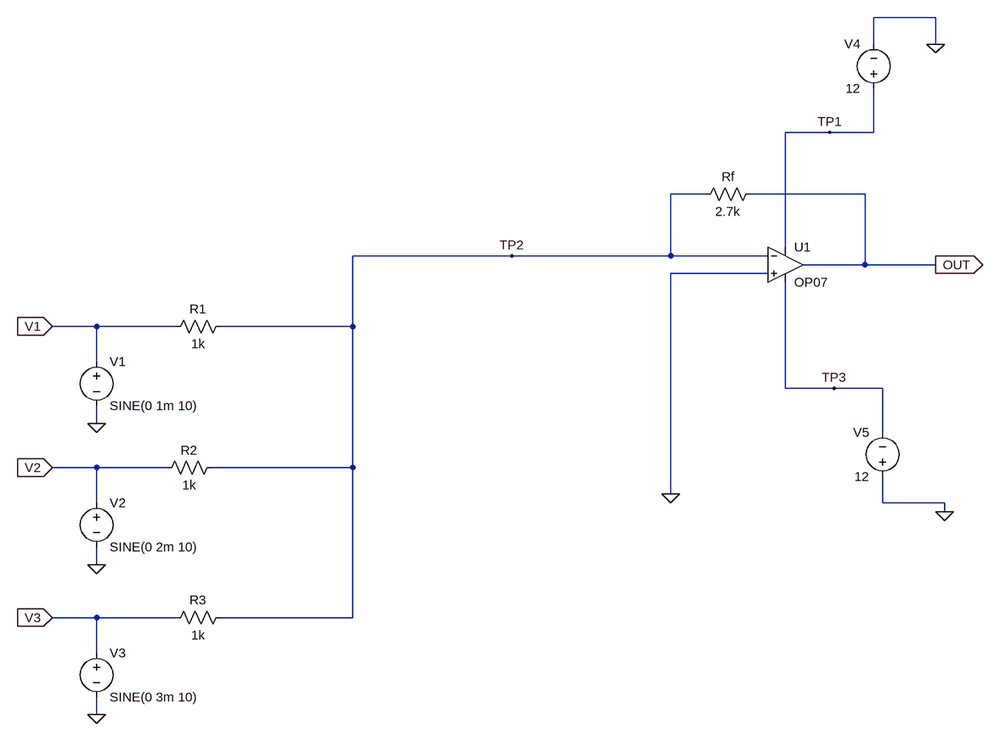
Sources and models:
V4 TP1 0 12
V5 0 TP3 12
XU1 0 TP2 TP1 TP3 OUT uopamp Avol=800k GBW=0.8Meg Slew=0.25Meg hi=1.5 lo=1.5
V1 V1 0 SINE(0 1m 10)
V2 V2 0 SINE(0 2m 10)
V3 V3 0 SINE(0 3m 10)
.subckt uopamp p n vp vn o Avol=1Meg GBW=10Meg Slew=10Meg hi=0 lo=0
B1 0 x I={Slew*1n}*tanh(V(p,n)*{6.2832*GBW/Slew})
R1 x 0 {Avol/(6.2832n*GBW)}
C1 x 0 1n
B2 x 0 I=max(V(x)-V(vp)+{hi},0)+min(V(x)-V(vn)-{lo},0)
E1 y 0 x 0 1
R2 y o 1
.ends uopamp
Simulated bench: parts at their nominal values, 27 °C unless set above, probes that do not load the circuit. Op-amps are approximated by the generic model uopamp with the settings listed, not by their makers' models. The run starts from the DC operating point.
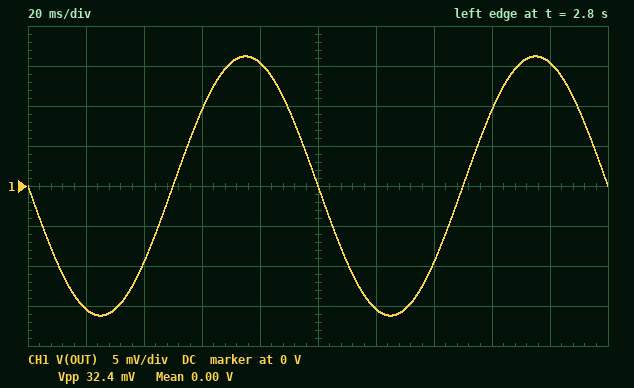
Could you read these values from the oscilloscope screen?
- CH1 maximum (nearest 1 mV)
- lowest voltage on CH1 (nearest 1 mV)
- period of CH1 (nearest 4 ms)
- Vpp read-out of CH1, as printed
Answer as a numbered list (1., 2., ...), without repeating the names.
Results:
1. 16 mV
2. -16 mV
3. 100 ms
4. 32.4 mV
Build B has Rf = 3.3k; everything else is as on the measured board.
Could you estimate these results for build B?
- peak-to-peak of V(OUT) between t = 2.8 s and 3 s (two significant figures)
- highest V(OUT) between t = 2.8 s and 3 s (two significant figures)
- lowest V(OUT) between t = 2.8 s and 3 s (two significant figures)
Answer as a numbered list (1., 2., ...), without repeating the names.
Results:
1. 40 mV
2. 20 mV
3. -20 mV
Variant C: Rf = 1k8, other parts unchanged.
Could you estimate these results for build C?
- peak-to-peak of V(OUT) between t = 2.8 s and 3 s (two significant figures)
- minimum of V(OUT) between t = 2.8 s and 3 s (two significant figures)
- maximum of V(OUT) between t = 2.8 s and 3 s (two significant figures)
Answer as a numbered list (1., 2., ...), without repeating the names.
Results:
1. 22 mV
2. -11 mV
3. 11 mV
